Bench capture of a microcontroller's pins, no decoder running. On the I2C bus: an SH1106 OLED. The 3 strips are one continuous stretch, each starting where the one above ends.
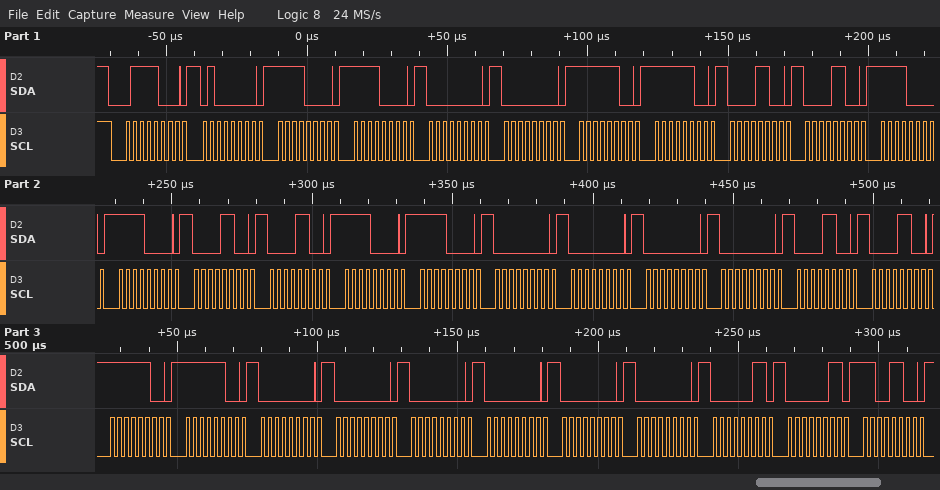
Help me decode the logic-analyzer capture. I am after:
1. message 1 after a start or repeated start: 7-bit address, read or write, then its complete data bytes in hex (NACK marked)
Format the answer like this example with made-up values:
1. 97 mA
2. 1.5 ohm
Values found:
1. 0x3C write: 40 F0 F0 00 00 FC FC 0C 0C F0 F0 0C 0C F0 F0 00 00 00 00 0C 0C FC FC 00 00 00 00 00 00 03 03 CC
